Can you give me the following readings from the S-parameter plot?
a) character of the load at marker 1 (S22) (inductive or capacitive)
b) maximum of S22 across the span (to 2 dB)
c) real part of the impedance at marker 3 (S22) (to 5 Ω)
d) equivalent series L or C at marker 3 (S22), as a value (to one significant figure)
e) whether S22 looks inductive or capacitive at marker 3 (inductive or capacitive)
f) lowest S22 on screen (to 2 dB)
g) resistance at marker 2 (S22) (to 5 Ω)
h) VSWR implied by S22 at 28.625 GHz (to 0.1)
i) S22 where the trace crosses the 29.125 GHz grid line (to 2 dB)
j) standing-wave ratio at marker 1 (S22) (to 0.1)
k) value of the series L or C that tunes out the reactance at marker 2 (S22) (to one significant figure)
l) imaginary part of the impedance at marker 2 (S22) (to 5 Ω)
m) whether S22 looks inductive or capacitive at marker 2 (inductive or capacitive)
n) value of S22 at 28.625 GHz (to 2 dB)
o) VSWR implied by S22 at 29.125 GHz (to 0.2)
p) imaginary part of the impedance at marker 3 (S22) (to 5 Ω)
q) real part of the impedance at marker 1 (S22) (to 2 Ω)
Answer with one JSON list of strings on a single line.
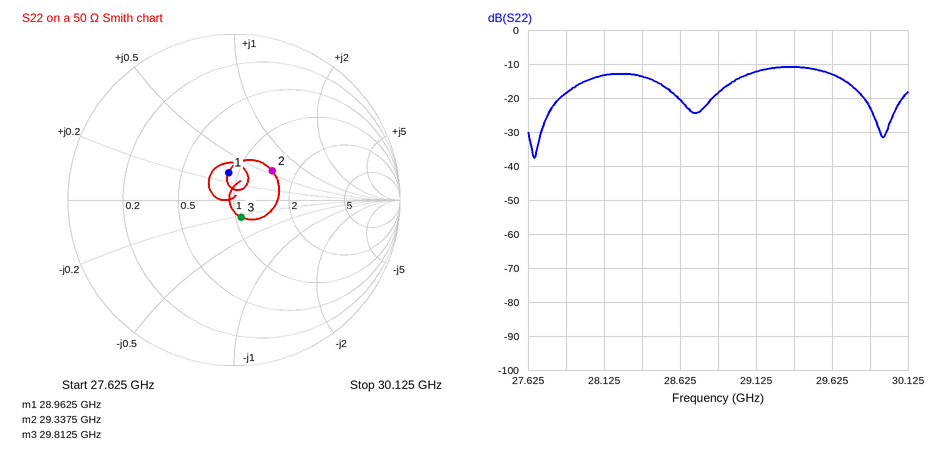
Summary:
["inductive", "-10 dB", "55 Ω", "500 fF", "capacitive", "-38 dB", "75 Ω", "1.2", "-12 dB", "1.4", "200 fF", "+30 Ω", "inductive", "-20 dB", "1.6", "-10 Ω", "44 Ω"]
